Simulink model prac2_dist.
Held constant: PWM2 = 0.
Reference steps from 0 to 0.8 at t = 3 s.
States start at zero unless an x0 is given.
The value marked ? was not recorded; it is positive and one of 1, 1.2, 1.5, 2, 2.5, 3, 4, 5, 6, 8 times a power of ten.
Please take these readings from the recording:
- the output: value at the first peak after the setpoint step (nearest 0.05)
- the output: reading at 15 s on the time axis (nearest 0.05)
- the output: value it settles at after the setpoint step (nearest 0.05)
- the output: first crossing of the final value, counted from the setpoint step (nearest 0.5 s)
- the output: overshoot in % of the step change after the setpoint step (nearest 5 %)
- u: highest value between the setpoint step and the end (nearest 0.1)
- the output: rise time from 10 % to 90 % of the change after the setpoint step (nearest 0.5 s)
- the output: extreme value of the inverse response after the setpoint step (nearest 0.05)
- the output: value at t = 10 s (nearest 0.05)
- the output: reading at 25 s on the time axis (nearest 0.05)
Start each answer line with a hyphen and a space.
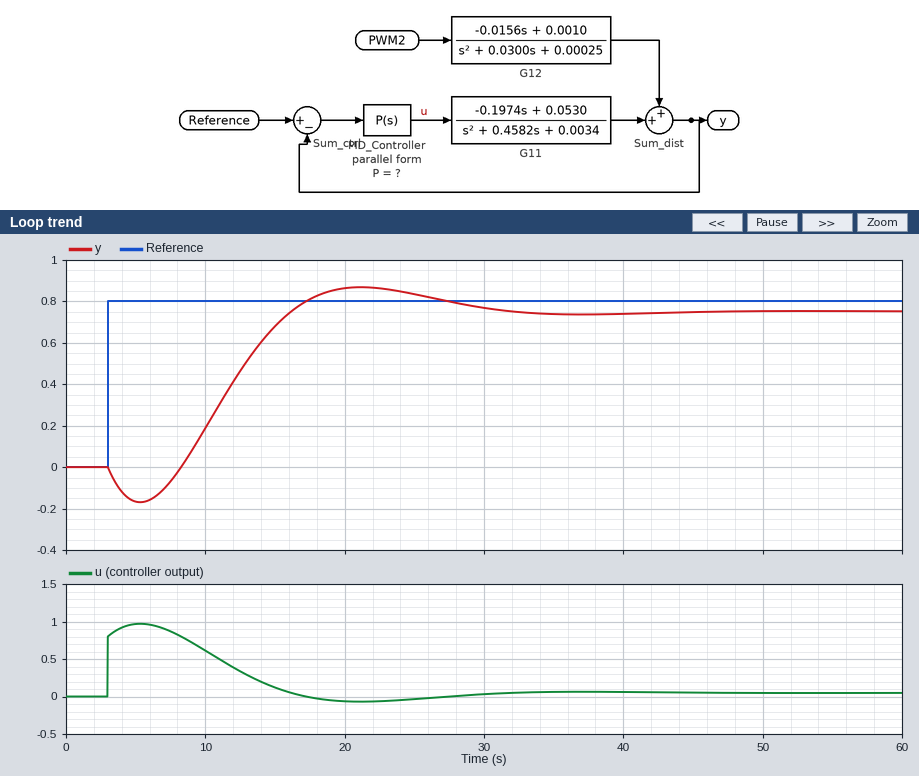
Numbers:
- 0.85
- 0.70
- 0.75
- 13.0 s
- 15 %
- 1.0
- 6.0 s
- -0.15
- 0.20
- 0.85
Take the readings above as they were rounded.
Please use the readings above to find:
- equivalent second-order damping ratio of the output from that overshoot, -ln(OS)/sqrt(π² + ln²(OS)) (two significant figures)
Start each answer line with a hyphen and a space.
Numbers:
- 0.52
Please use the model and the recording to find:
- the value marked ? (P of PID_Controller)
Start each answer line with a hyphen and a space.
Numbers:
- 1
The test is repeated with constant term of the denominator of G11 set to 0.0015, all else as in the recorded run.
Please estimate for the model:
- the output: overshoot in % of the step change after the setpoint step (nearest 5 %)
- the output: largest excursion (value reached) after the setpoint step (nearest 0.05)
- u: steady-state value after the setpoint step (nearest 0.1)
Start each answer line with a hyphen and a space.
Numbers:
- 15 %
- 0.90
- 0.0
